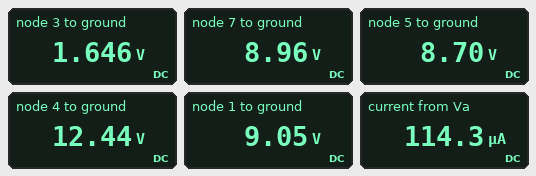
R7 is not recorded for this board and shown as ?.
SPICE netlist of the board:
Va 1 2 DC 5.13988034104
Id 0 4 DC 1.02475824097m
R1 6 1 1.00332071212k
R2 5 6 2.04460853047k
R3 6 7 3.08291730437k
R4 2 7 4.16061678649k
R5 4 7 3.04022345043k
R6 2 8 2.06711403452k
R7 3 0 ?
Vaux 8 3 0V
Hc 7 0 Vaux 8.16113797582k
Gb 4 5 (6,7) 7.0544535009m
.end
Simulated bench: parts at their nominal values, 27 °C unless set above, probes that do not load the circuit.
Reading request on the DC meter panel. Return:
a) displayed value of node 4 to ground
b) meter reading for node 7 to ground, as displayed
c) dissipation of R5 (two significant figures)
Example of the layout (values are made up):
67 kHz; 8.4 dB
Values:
12.44 V; 8.96 V; 4.0 mW
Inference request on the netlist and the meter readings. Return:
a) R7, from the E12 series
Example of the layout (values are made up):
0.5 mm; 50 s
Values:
1.5 kΩ
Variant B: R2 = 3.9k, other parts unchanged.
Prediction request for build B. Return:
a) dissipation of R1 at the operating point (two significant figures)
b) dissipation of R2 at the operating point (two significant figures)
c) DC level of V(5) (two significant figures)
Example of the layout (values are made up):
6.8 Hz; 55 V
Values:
13 µW; 56 µW; 8.5 V
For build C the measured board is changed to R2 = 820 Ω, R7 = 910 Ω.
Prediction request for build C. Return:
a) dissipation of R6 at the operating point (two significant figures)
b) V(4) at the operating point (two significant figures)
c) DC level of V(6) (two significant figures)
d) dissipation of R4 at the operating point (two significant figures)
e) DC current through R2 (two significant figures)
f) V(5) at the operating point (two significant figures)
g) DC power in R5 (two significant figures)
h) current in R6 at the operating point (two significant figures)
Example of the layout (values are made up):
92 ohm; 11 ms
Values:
1.9 mW; 12 V; 7.7 V; 5.9 mW; 250 µA; 7.5 V; 4.9 mW; 950 µA
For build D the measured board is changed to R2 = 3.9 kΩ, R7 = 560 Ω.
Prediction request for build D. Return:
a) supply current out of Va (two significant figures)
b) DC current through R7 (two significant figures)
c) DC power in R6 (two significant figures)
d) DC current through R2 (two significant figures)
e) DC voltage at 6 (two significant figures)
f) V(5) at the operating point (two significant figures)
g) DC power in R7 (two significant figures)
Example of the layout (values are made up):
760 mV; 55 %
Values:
290 µA; 880 µA; 1.6 mW; 310 µA; 7.2 V; 6.0 V; 440 µW
